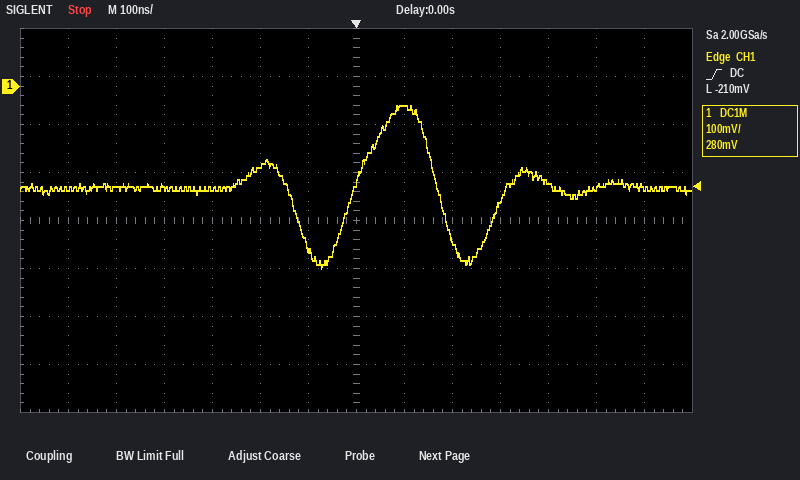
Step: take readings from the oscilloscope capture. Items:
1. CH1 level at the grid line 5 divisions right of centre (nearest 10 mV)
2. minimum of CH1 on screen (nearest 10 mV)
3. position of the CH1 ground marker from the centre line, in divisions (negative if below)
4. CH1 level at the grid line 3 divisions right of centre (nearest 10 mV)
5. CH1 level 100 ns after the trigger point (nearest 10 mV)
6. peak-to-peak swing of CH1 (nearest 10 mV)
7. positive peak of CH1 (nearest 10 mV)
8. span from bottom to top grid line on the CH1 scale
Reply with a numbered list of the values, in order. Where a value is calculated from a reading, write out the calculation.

1. -210 mV
2. -380 mV
3. +2.8 div
4. -240 mV
5. -40 mV
6. -40 mV − (-380 mV) = 340 mV
7. -40 mV
8. 800 mV
